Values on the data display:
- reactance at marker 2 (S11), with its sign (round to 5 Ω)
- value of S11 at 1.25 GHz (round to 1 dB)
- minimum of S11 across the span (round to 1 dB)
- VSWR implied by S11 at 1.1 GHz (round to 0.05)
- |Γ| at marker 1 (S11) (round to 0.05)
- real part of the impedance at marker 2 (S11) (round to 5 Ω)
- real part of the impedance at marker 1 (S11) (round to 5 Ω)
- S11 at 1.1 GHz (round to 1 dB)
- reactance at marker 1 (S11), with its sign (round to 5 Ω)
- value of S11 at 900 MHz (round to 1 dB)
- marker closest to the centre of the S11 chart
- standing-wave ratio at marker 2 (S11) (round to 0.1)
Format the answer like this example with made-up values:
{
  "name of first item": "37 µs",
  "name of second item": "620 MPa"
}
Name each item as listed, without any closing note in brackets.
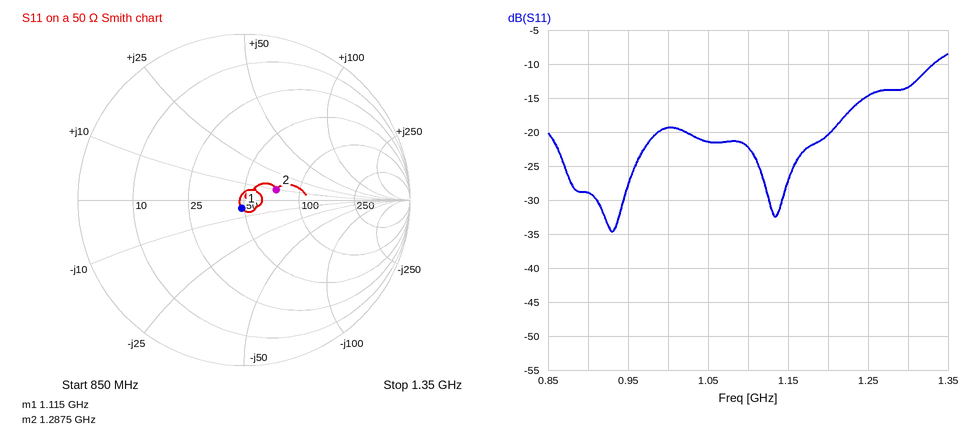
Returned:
{
  "reactance at marker 2 (S11), with its sign": "+10 Ω",
  "value of S11 at 1.25 GHz": "-15 dB",
  "minimum of S11 across the span": "-35 dB",
  "VSWR implied by S11 at 1.1 GHz": "1.15",
  "|Γ| at marker 1 (S11)": "0.05",
  "real part of the impedance at marker 2 (S11)": "75 Ω",
  "real part of the impedance at marker 1 (S11)": "50 Ω",
  "S11 at 1.1 GHz": "-22 dB",
  "reactance at marker 1 (S11), with its sign": "-5 Ω",
  "value of S11 at 900 MHz": "-29 dB",
  "marker closest to the centre of the S11 chart": "marker 1",
  "standing-wave ratio at marker 2 (S11)": "1.5"
}
